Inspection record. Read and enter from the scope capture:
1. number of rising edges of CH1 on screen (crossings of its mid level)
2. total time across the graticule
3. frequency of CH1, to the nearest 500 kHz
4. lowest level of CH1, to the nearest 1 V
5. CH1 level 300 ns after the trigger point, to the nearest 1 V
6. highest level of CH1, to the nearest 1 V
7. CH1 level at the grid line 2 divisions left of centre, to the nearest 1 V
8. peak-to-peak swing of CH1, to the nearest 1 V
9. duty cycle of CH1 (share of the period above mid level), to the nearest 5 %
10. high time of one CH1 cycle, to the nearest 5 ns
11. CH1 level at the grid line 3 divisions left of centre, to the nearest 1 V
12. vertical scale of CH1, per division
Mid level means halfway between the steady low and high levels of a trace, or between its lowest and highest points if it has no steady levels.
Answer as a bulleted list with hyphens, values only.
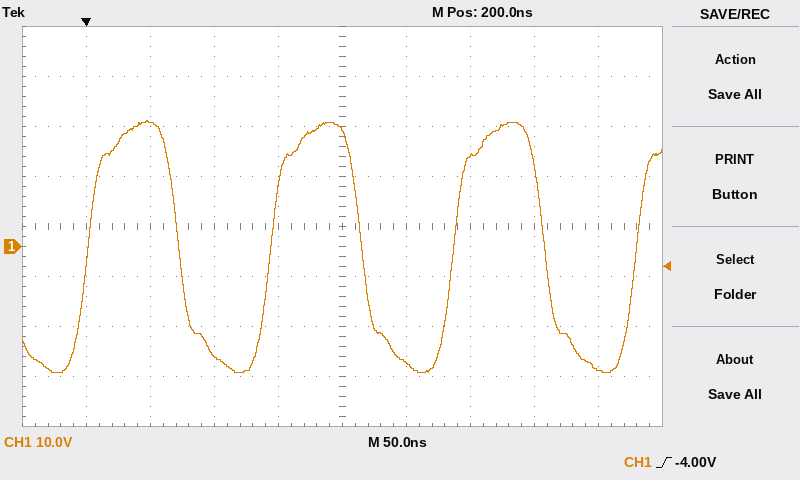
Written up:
- 4
- 500 ns
- 7.0 MHz
- -25 V
- 18 V
- 25 V
- -22 V
- 50 V
- 50 %
- 70 ns
- 25 V
- 10 V
